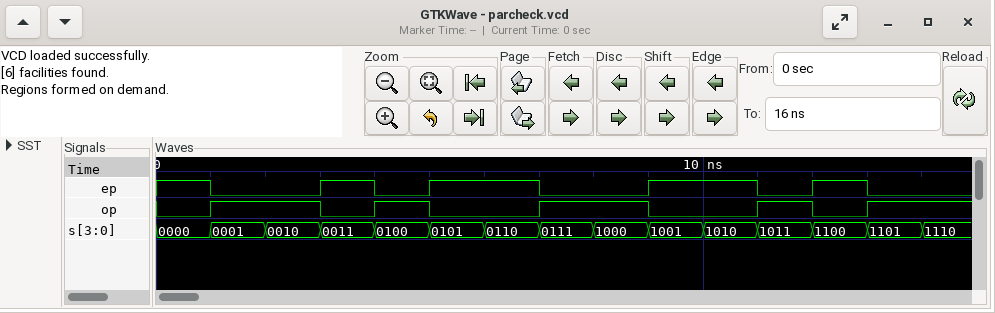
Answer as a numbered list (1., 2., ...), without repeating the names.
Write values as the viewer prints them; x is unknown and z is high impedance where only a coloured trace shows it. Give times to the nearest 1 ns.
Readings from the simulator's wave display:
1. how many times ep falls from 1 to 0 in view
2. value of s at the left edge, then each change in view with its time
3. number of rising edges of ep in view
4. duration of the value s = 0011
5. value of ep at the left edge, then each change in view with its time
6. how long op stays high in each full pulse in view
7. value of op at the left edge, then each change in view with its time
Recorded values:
1. 5
2. 0000, 0001 at 1 ns, 0010 at 2 ns, 0011 at 3 ns, 0100 at 4 ns, 0101 at 5 ns, 0110 at 6 ns, 0111 at 7 ns, 1000 at 8 ns, 1001 at 9 ns, 1010 at 10 ns, 1011 at 11 ns, 1100 at 12 ns, 1101 at 13 ns, 1110 at 14 ns
3. 4
4. 1 ns
5. 1, 0 at 1 ns, 1 at 3 ns, 0 at 4 ns, 1 at 5 ns, 0 at 7 ns, 1 at 9 ns, 0 at 11 ns, 1 at 12 ns, 0 at 13 ns
6. 2 ns, 1 ns, 2 ns, 1 ns
7. 0, 1 at 1 ns, 0 at 3 ns, 1 at 4 ns, 0 at 5 ns, 1 at 7 ns, 0 at 9 ns, 1 at 11 ns, 0 at 12 ns, 1 at 13 ns
